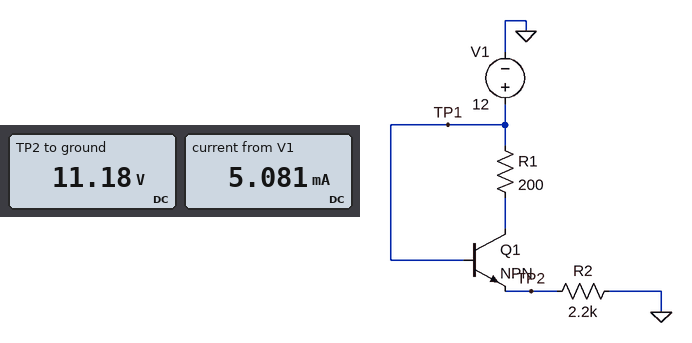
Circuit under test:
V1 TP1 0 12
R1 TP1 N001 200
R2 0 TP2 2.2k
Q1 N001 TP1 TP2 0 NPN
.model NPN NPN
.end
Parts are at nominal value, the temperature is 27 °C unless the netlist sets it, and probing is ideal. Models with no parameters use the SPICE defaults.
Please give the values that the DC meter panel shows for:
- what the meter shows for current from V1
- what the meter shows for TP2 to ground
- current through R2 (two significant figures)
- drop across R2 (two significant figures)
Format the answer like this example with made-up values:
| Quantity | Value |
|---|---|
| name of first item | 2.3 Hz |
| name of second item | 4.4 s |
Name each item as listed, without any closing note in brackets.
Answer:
| Quantity | Value |
|---|---|
| what the meter shows for current from V1 | 5.081 mA |
| what the meter shows for TP2 to ground | 11.18 V |
| current through R2 | 5.1 mA |
| drop across R2 | 11 V |
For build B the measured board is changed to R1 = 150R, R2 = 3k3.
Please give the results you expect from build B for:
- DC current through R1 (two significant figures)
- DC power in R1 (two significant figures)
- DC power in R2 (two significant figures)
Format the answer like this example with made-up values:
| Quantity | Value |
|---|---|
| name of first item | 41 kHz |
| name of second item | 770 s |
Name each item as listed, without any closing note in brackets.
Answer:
| Quantity | Value |
|---|---|
| DC current through R1 | 3.4 mA |
| DC power in R1 | 1.7 mW |
| DC power in R2 | 38 mW |
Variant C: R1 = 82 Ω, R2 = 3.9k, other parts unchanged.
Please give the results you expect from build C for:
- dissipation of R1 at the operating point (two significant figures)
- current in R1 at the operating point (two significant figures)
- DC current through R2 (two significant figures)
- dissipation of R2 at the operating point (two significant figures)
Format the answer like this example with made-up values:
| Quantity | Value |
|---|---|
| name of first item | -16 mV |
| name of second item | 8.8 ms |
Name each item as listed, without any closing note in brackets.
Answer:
| Quantity | Value |
|---|---|
| dissipation of R1 at the operating point | 660 µW |
| current in R1 at the operating point | 2.8 mA |
| DC current through R2 | 2.9 mA |
| dissipation of R2 at the operating point | 32 mW |
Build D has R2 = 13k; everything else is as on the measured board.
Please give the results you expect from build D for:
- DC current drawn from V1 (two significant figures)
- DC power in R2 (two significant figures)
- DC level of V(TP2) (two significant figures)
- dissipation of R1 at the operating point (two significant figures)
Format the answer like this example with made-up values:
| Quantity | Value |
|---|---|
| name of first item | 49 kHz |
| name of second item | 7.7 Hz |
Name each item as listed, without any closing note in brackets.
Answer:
| Quantity | Value |
|---|---|
| DC current drawn from V1 | 860 µA |
| DC power in R2 | 9.7 mW |
| DC level of V(TP2) | 11 V |
| dissipation of R1 at the operating point | 150 µW |
